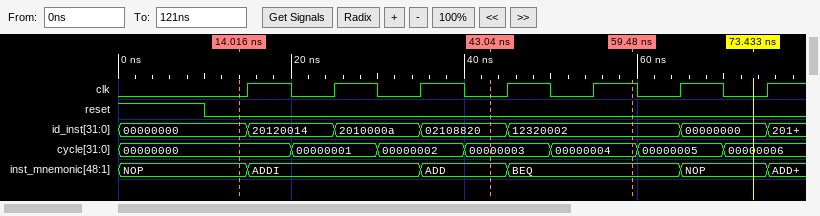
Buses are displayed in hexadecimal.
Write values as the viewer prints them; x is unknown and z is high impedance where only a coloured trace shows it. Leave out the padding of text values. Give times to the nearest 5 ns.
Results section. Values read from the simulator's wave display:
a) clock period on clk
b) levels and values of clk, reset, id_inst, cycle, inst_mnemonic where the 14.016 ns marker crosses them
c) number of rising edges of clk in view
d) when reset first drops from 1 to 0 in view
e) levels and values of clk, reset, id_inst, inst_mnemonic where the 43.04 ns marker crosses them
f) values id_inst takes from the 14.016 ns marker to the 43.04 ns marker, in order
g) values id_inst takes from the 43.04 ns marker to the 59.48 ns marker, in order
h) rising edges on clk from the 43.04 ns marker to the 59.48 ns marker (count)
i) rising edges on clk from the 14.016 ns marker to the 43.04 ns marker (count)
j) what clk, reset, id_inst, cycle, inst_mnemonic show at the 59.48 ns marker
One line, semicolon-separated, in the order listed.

10 ns; clk=0, reset=0, id_inst=00000000, cycle=00000000, inst_mnemonic=NOP; 7; 10 ns; clk=0, reset=0, id_inst=02108820, inst_mnemonic=ADD; 00000000, 20120014, 2010000a, 02108820; 02108820, 12320002; 2; 3; clk=1, reset=0, id_inst=12320002, cycle=00000004, inst_mnemonic=BEQ
